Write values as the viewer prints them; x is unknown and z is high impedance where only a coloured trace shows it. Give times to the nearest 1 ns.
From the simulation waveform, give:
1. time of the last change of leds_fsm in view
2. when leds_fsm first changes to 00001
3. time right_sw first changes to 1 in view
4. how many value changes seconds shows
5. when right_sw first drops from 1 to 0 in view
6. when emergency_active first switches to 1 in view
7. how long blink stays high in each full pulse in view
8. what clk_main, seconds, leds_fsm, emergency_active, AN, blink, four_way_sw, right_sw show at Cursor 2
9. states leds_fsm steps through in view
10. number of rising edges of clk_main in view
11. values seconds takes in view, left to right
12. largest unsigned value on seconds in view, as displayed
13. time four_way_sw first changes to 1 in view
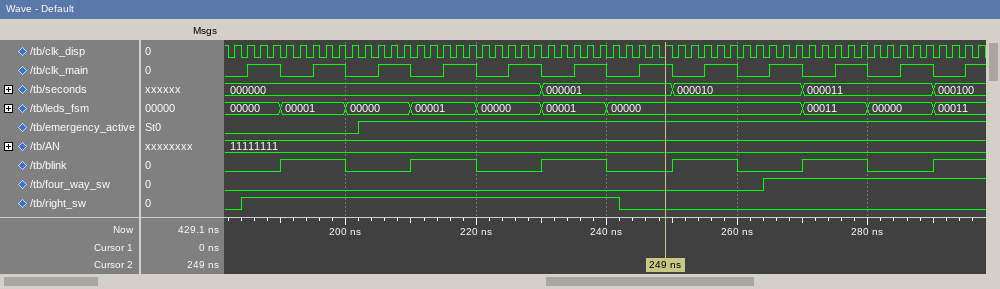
290 ns
190 ns
184 ns
4
242 ns
202 ns
10 ns, 10 ns, 10 ns, 10 ns, 10 ns
clk_main=1, seconds=000001, leds_fsm=00000, emergency_active=1, AN=11111111, blink=0, four_way_sw=0, right_sw=0
00000, 00001, 00000, 00001, 00000, 00001, 00000, 00011, 00000, 00011
12
000000, 000001, 000010, 000011, 000100
000100
264 ns
